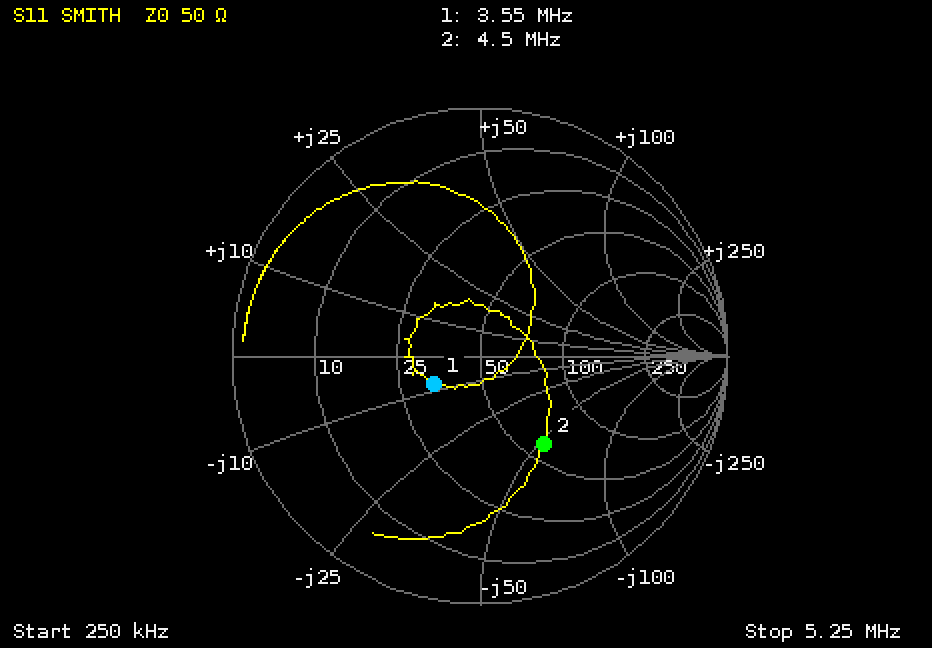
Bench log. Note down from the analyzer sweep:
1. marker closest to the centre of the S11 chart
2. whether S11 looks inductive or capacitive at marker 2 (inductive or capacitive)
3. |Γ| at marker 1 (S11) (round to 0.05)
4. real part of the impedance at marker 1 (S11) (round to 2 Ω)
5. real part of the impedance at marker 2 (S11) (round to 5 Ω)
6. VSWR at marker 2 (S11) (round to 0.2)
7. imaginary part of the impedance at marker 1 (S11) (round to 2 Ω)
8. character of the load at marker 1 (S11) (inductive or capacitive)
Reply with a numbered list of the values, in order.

1. marker 1
2. capacitive
3. 0.20
4. 34 Ω
5. 60 Ω
6. 2.6
7. -8 Ω
8. capacitive
